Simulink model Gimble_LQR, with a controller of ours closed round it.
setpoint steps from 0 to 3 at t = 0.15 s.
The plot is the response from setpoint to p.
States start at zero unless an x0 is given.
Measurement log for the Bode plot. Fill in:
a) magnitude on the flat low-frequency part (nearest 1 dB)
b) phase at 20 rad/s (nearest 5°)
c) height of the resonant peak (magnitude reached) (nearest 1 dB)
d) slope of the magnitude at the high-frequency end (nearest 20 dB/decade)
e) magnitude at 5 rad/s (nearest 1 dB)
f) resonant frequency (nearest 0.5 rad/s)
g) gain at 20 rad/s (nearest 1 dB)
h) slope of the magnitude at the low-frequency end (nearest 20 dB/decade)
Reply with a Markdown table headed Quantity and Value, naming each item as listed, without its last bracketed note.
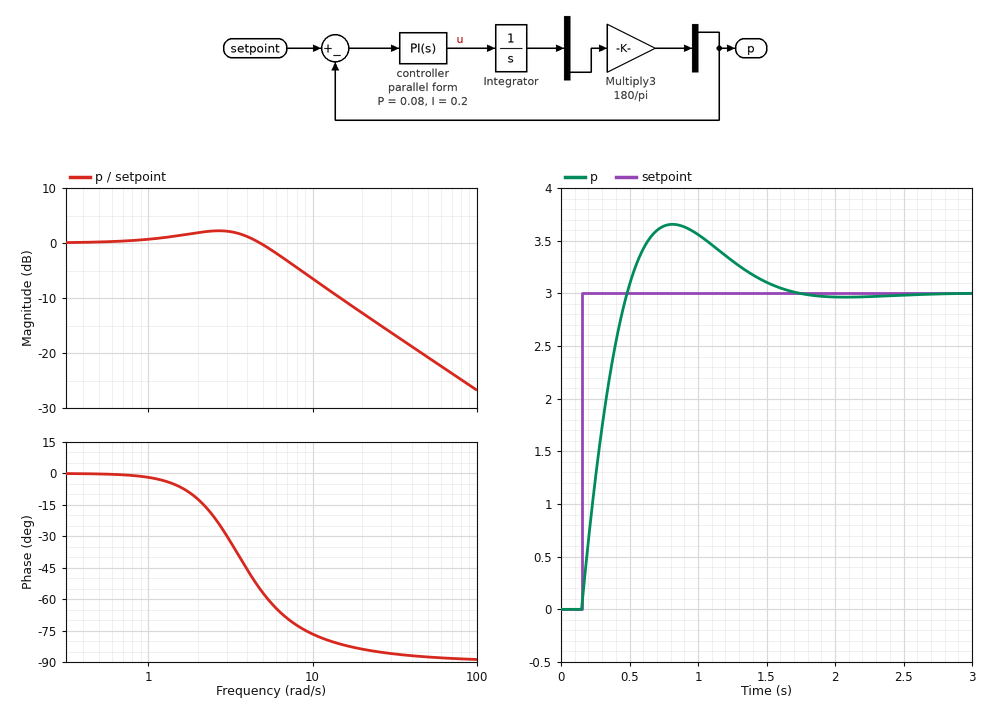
| Quantity | Value |
|---|---|
| magnitude on the flat low-frequency part | 0 dB |
| phase at 20 rad/s | -85° |
| height of the resonant peak (magnitude reached) | 2 dB |
| slope of the magnitude at the high-frequency end | -20 dB/decade |
| magnitude at 5 rad/s | 0 dB |
| resonant frequency | 2.5 rad/s |
| gain at 20 rad/s | -13 dB |
| slope of the magnitude at the low-frequency end | 0 dB/decade |
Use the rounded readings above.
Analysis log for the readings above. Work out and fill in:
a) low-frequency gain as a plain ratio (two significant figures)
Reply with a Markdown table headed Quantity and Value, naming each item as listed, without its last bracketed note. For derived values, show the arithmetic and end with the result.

| Quantity | Value |
|---|---|
| low-frequency gain as a plain ratio | 10^(0 / 20) = 1.0 |
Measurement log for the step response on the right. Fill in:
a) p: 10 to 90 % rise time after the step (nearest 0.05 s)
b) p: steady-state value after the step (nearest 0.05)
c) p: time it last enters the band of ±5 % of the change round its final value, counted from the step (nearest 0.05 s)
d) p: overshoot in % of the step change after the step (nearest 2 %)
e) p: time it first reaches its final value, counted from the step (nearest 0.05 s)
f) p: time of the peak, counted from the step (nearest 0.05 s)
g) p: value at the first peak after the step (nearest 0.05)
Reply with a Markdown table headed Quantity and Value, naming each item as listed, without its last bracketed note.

| Quantity | Value |
|---|---|
| p: 10 to 90 % rise time after the step | 0.25 s |
| p: steady-state value after the step | 3.00 |
| p: time it last enters the band of ±5 % of the change round its final value, counted from the step | 1.30 s |
| p: overshoot in % of the step change after the step | 22 % |
| p: time it first reaches its final value, counted from the step | 0.35 s |
| p: time of the peak, counted from the step | 0.65 s |
| p: value at the first peak after the step | 3.65 |
